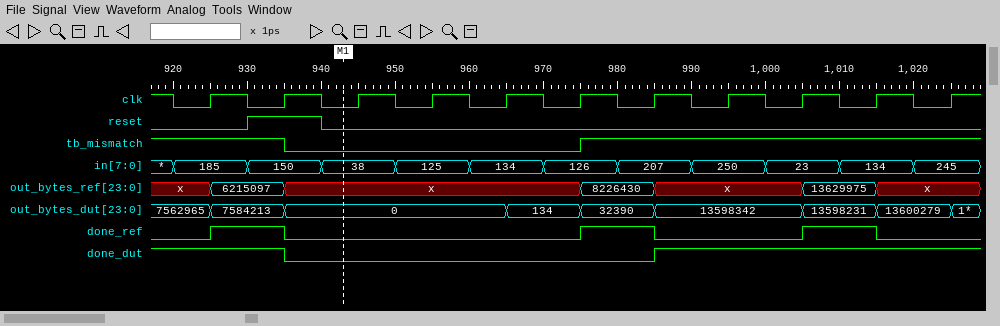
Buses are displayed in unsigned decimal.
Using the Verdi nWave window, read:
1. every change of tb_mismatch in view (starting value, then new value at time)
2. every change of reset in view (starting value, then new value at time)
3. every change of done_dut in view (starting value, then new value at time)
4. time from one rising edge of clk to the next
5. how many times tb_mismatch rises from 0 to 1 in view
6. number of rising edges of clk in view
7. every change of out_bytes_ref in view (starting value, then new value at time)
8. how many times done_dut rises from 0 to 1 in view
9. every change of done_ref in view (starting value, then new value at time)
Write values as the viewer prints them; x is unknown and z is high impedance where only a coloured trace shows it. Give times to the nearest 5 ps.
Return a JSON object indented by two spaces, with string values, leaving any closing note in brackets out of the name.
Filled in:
{
  "every change of tb_mismatch in view": "1, 0 at 935 ps, 1 at 975 ps",
  "every change of reset in view": "0, 1 at 930 ps, 0 at 940 ps",
  "every change of done_dut in view": "1, 0 at 935 ps, 1 at 985 ps",
  "time from one rising edge of clk to the next": "10 ps",
  "how many times tb_mismatch rises from 0 to 1 in view": "1",
  "number of rising edges of clk in view": "11",
  "every change of out_bytes_ref in view": "x, 6215097 at 925 ps, x at 935 ps, 8226430 at 975 ps, x at 985 ps, 13629975 at 1005 ps, x at 1015 ps",
  "how many times done_dut rises from 0 to 1 in view": "1",
  "every change of done_ref in view": "0, 1 at 925 ps, 0 at 935 ps, 1 at 975 ps, 0 at 985 ps, 1 at 1005 ps, 0 at 1015 ps"
}
